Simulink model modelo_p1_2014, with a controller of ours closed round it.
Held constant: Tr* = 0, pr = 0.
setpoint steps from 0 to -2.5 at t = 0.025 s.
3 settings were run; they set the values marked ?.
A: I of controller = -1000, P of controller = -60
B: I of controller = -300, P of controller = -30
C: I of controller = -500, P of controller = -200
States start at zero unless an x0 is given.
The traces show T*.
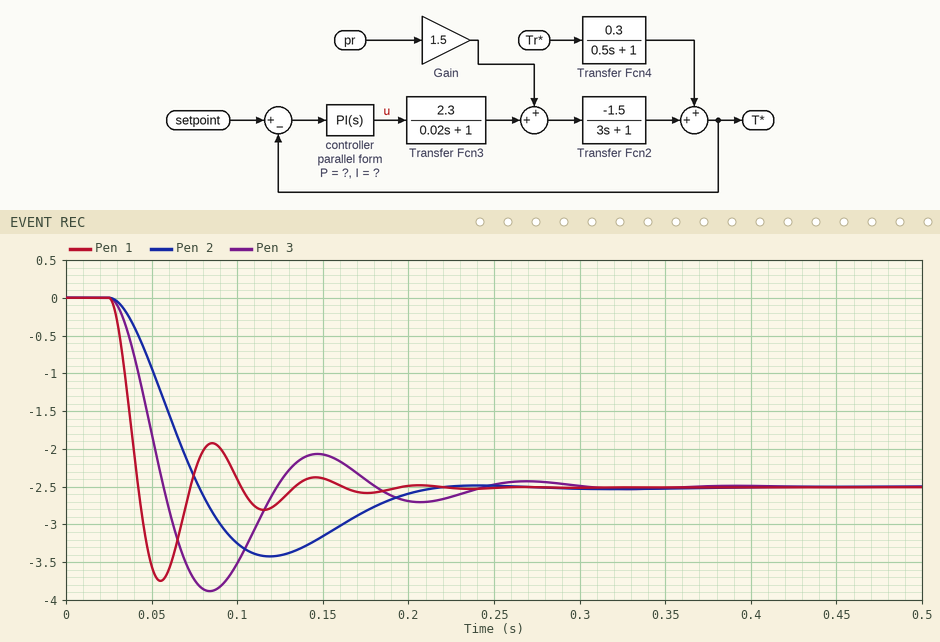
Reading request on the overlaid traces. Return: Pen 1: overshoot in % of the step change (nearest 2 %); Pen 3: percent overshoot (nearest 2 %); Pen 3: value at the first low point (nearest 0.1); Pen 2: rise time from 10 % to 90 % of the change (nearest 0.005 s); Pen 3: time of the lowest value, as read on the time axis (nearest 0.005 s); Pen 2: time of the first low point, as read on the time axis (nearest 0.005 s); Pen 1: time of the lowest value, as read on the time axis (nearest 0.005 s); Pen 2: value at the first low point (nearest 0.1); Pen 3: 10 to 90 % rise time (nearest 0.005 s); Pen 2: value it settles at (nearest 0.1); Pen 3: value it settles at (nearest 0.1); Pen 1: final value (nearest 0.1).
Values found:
50 %
56 %
-3.9
0.035 s
0.085 s
0.120 s
0.055 s
-3.4
0.020 s
-2.5
-2.5
-2.5
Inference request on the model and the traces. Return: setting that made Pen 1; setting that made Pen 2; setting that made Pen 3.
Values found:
C
B
A
